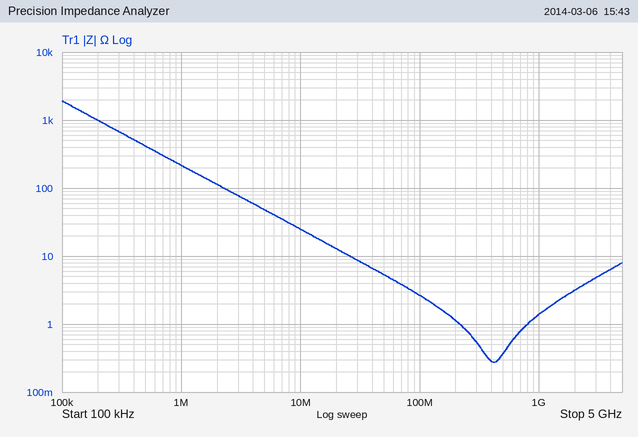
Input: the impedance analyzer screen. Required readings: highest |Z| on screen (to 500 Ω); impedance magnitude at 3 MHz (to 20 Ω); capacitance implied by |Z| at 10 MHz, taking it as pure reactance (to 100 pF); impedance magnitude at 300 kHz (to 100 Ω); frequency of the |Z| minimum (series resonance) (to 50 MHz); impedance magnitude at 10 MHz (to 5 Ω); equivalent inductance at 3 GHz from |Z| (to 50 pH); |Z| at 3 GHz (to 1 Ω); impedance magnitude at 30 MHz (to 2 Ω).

2.0 kΩ
80 Ω
600 pF
700 Ω
400 MHz
25 Ω
250 pH
5 Ω
8 Ω
